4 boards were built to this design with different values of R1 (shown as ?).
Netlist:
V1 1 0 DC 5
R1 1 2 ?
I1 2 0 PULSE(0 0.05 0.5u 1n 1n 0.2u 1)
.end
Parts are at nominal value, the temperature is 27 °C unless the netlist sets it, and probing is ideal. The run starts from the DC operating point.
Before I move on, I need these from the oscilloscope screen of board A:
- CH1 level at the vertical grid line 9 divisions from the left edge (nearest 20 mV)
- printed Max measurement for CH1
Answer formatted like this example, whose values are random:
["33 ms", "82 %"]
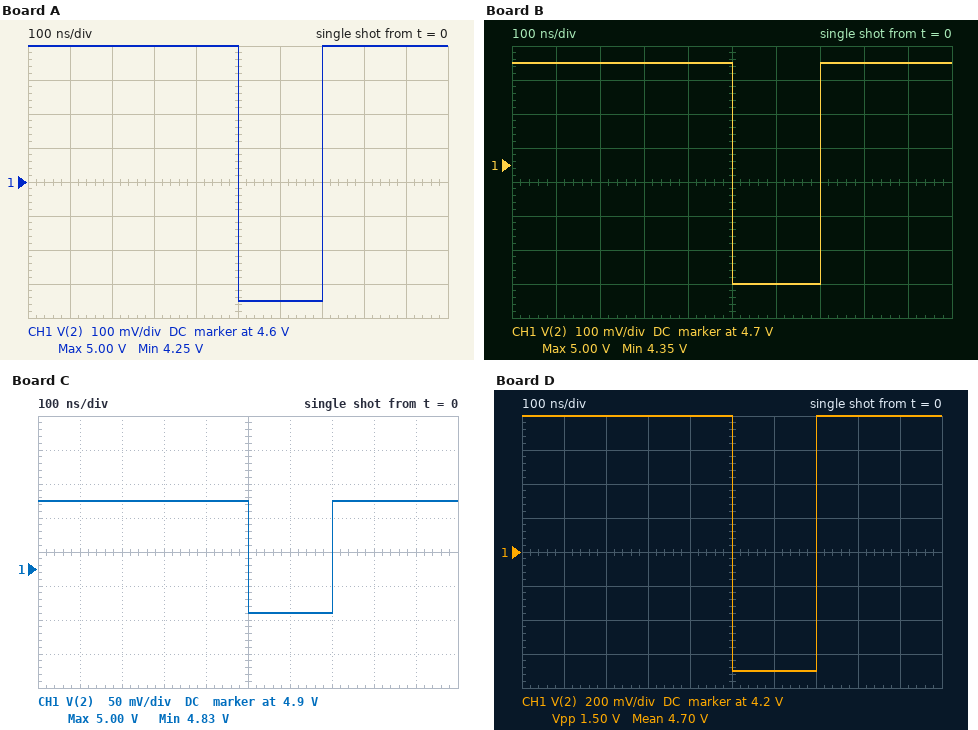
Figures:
["5.00 V", "5.00 V"]
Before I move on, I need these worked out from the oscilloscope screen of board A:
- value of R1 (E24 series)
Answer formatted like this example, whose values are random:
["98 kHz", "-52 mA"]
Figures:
["15 Ω"]
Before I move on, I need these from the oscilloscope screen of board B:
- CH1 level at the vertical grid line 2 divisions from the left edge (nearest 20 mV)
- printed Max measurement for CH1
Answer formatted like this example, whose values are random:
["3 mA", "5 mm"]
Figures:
["5.00 V", "5.00 V"]
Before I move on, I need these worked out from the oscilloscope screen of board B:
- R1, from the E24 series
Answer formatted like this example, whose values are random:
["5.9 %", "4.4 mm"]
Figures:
["13 Ω"]
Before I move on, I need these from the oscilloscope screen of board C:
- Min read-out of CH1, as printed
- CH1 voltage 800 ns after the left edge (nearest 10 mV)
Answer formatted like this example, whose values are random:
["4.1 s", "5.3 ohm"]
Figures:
["4.83 V", "5.00 V"]
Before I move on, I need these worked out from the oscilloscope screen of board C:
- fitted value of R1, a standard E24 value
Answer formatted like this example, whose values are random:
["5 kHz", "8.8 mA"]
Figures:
["3.3 Ω"]
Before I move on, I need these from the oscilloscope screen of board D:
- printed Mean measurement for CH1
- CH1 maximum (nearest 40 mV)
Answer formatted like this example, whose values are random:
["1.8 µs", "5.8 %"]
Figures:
["4.70 V", "5.00 V"]
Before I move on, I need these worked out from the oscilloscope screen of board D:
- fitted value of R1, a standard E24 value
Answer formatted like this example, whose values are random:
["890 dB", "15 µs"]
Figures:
["30 Ω"]
